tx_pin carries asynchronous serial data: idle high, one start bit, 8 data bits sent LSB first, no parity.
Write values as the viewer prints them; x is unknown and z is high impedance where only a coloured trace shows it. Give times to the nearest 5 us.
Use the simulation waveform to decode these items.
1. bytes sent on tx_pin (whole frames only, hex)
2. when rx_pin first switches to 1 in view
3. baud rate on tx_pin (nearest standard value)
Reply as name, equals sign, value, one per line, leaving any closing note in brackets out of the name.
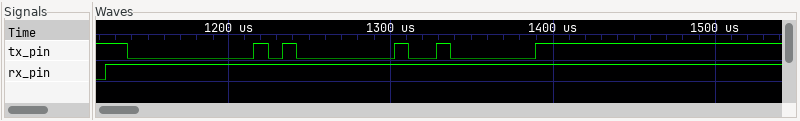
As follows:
bytes sent on tx_pin = 00, 01, 02
when rx_pin first switches to 1 in view = 1125 us
baud rate on tx_pin = 115200 baud
